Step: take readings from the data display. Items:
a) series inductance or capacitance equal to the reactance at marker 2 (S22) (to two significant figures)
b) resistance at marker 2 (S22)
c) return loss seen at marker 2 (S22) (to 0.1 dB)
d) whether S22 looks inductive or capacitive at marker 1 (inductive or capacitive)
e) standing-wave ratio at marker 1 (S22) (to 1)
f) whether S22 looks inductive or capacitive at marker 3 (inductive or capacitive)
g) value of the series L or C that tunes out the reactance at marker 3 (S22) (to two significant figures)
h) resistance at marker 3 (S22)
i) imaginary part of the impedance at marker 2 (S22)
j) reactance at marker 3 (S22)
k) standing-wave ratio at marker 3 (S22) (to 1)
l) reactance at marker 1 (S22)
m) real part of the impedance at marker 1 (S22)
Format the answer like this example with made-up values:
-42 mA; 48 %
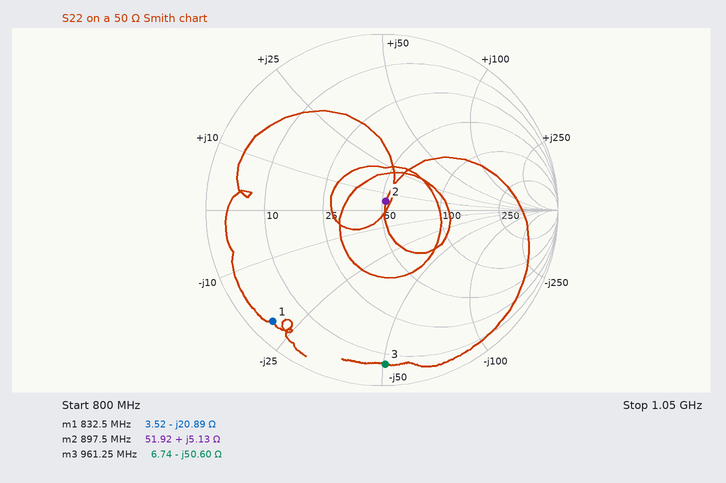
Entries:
910 pH; 51.92 Ω; 25.4 dB; capacitive; 17; capacitive; 8.4 nH; 6.74 Ω; +5.13 Ω; -50.60 Ω; 15; -20.89 Ω; 3.52 Ω
